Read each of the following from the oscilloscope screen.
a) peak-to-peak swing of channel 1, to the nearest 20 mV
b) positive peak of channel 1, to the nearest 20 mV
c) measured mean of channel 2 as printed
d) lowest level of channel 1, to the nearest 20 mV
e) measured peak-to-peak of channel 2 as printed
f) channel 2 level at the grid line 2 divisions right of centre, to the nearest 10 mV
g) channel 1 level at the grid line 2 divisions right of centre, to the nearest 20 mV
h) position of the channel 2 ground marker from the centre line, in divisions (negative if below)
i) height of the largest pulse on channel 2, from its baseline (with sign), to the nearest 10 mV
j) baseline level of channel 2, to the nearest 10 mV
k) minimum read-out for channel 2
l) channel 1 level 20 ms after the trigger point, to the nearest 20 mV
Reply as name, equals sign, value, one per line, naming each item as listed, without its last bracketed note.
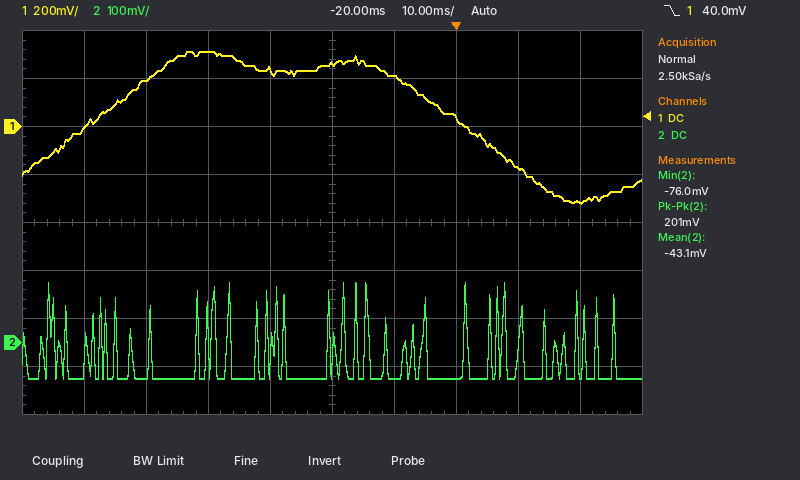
peak-to-peak swing of channel 1, to the nearest 20 mV = 640 mV
positive peak of channel 1, to the nearest 20 mV = 320 mV
measured mean of channel 2 as printed = -43.1 mV
lowest level of channel 1, to the nearest 20 mV = -320 mV
measured peak-to-peak of channel 2 as printed = 201 mV
channel 2 level at the grid line 2 divisions right of centre, to the nearest 10 mV = -80 mV
channel 1 level at the grid line 2 divisions right of centre, to the nearest 20 mV = 40 mV
position of the channel 2 ground marker from the centre line, in divisions = -2.5 div
height of the largest pulse on channel 2, from its baseline (with sign), to the nearest 10 mV = +200 mV
baseline level of channel 2, to the nearest 10 mV = -80 mV
minimum read-out for channel 2 = -76.0 mV
channel 1 level 20 ms after the trigger point, to the nearest 20 mV = -320 mV
